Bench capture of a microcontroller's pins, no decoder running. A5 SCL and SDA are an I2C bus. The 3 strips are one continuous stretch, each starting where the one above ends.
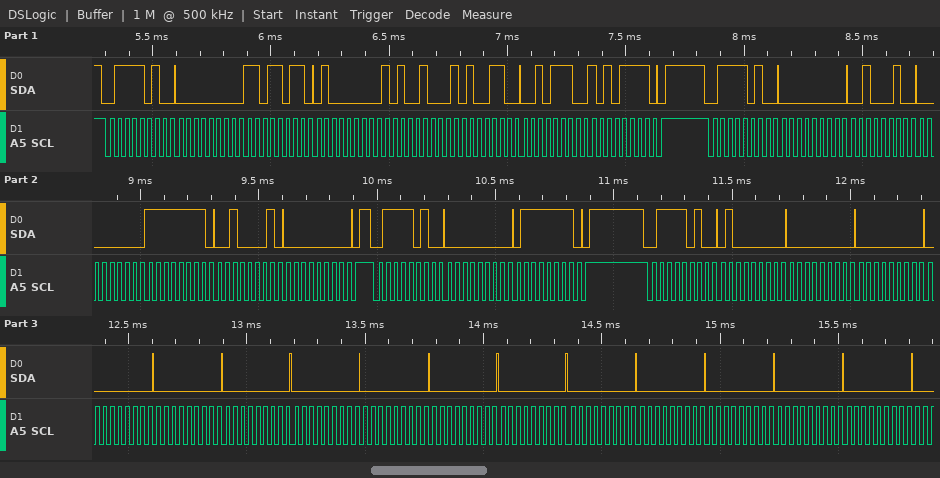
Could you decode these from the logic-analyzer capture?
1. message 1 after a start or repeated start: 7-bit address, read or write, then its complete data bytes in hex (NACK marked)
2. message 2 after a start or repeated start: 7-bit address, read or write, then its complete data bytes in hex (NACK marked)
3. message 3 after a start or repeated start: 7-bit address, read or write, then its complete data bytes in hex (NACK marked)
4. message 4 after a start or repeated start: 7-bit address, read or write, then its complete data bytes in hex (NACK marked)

0x3D write: 00 DB 40 A4 A6 2E AF
0x3D write: 00 22 00 FF 21 00
0x3D write: 00 7F
0x3D write: 40 00 00 00 00 00 00 00 00 00 00 00 00 00 00
